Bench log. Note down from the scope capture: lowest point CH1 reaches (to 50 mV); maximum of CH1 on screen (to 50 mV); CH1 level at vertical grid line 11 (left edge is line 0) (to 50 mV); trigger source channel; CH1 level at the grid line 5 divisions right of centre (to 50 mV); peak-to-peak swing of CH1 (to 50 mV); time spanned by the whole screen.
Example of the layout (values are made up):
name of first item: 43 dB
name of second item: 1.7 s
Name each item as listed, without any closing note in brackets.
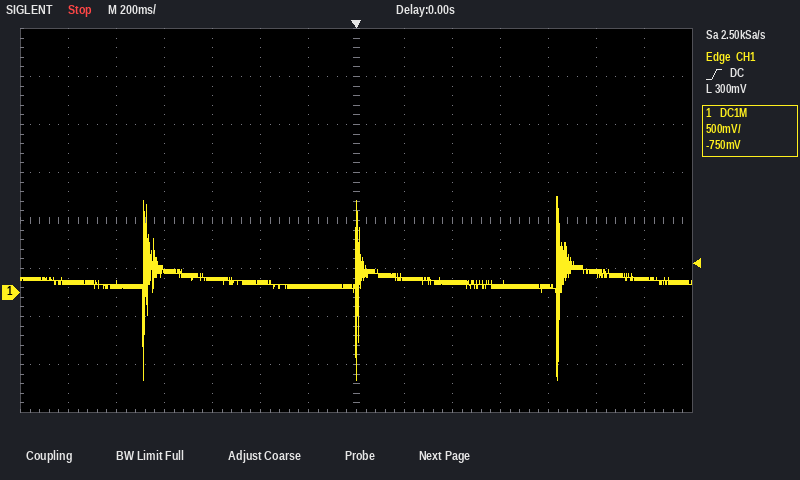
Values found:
lowest point CH1 reaches: -900 mV
maximum of CH1 on screen: 1.00 V
CH1 level at vertical grid line 11 (left edge is line 0): 50 mV
trigger source channel: CH1
CH1 level at the grid line 5 divisions right of centre: 200 mV
peak-to-peak swing of CH1: 1.90 V
time spanned by the whole screen: 2.8 s
